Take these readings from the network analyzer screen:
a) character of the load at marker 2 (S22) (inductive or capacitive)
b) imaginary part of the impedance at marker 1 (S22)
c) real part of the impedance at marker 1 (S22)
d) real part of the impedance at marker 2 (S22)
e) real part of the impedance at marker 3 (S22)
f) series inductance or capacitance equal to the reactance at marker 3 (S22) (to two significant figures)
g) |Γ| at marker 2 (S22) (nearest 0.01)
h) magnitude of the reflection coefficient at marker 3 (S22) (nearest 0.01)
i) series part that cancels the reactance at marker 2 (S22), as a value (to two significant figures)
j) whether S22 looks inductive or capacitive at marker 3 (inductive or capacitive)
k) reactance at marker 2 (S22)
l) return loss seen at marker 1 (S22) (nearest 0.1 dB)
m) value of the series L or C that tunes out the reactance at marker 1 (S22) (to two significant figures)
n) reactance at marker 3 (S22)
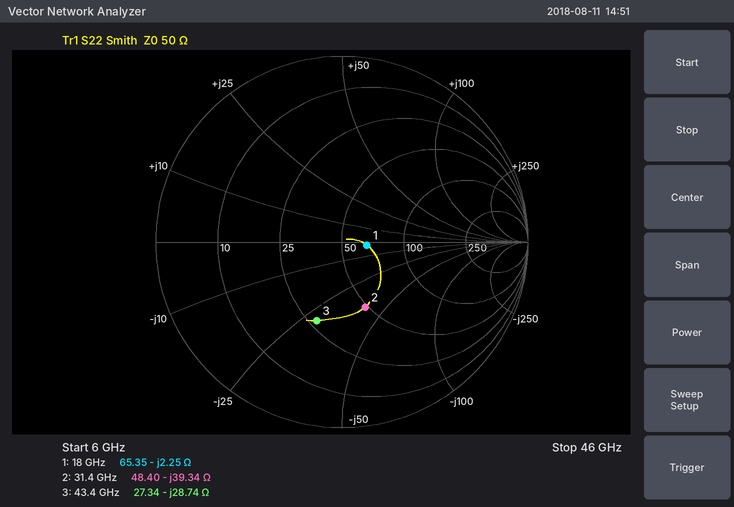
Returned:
capacitive
-2.25 Ω
65.35 Ω
48.40 Ω
27.34 Ω
130 fF
0.37
0.44
200 pH
capacitive
-39.34 Ω
17.4 dB
20 pH
-28.74 Ω
